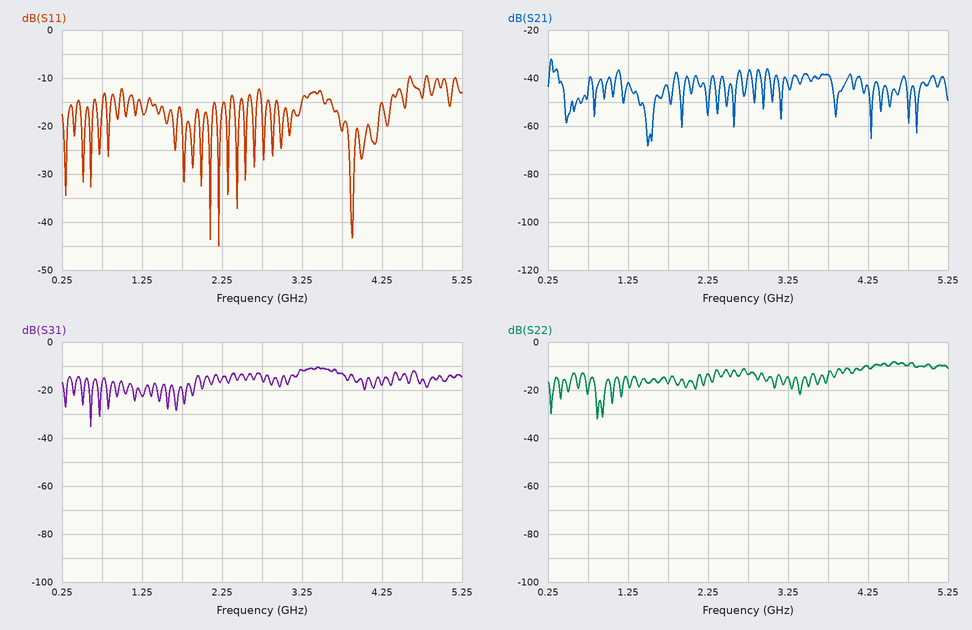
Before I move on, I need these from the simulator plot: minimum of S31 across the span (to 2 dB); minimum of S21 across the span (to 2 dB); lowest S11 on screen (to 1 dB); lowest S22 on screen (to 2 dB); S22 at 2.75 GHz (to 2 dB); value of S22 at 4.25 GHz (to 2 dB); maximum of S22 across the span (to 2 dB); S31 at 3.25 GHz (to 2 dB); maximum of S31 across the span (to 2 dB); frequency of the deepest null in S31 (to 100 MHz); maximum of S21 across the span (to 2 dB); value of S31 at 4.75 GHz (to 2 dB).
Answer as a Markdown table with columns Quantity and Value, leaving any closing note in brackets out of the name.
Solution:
| Quantity | Value |
|---|---|
| minimum of S31 across the span | -36 dB |
| minimum of S21 across the span | -68 dB |
| lowest S11 on screen | -45 dB |
| lowest S22 on screen | -32 dB |
| S22 at 2.75 GHz | -14 dB |
| value of S22 at 4.25 GHz | -10 dB |
| maximum of S22 across the span | -8 dB |
| S31 at 3.25 GHz | -12 dB |
| maximum of S31 across the span | -10 dB |
| frequency of the deepest null in S31 | 600 MHz |
| maximum of S21 across the span | -32 dB |
| value of S31 at 4.75 GHz | -16 dB |
